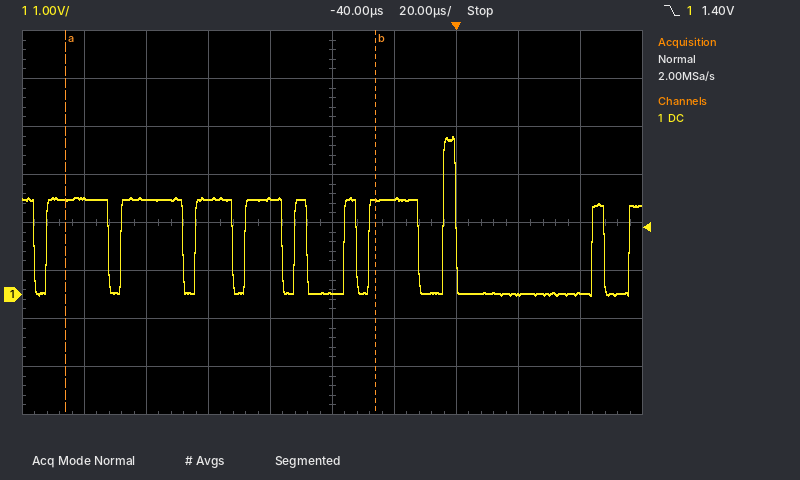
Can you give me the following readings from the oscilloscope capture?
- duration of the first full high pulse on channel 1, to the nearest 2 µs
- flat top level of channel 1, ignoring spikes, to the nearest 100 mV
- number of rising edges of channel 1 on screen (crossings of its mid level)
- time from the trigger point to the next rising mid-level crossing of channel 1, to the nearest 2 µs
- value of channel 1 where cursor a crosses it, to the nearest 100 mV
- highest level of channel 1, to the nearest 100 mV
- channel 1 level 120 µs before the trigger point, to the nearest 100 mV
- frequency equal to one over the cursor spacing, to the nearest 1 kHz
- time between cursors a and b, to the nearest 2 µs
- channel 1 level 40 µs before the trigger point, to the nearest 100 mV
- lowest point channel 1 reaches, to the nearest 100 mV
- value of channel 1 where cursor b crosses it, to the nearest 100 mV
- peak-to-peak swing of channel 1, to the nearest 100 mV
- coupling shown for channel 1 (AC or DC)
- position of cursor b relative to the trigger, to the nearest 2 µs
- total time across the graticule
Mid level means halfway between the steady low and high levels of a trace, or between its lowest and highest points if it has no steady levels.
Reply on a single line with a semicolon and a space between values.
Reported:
20 µs; 2.0 V; 10; 44 µs; 2.0 V; 3.3 V; 2.0 V; 10 kHz; 100 µs; 0.0 V; 0.0 V; 2.0 V; 3.3 V; DC; -26 µs; 200 µs
